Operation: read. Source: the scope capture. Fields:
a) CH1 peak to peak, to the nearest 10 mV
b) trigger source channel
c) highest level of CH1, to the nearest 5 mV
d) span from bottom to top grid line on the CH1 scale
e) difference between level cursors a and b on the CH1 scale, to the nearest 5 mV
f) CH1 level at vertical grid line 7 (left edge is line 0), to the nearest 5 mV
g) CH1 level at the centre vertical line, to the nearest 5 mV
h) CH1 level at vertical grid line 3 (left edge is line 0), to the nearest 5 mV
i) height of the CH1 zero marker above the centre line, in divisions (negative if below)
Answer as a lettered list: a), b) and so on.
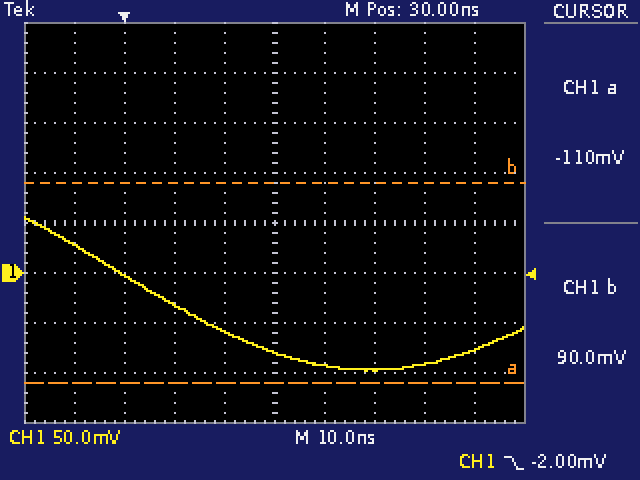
a) 150 mV
b) CH1
c) 55 mV
d) 400 mV
e) 200 mV
f) -95 mV
g) -80 mV
h) -30 mV
i) -1.0 div
